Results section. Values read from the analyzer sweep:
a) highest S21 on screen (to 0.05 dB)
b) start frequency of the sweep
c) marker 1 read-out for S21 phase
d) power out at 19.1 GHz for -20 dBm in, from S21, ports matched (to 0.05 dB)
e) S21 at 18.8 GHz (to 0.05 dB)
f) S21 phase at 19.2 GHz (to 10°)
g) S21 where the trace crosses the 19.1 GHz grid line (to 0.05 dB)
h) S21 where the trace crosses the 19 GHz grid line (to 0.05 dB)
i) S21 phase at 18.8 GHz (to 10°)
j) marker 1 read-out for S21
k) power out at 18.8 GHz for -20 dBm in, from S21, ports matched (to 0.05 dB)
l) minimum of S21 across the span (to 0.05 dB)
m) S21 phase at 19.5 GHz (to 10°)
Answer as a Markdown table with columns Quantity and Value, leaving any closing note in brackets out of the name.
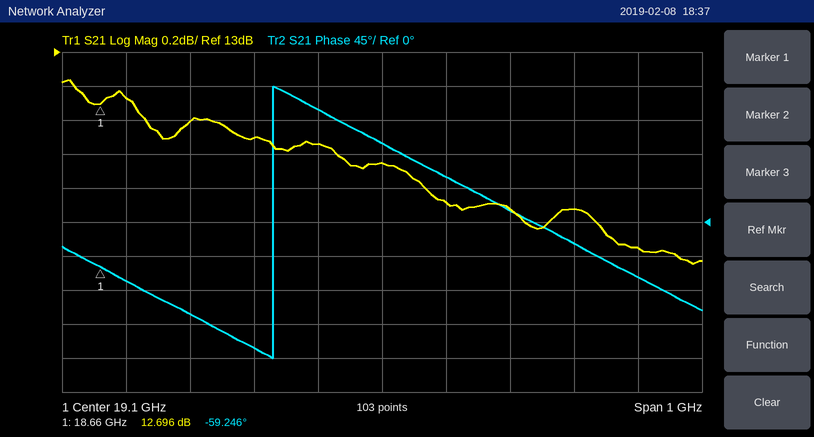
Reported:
| Quantity | Value |
|---|---|
| highest S21 on screen | 12.85 dB |
| start frequency of the sweep | 18.6 GHz |
| marker 1 read-out for S21 phase | -59.246° |
| power out at 19.1 GHz for -20 dBm in, from S21, ports matched | -7.65 dBm |
| S21 at 18.8 GHz | 12.60 dB |
| S21 phase at 19.2 GHz | 60° |
| S21 where the trace crosses the 19.1 GHz grid line | 12.35 dB |
| S21 where the trace crosses the 19 GHz grid line | 12.45 dB |
| S21 phase at 18.8 GHz | -120° |
| marker 1 read-out for S21 | 12.696 dB |
| power out at 18.8 GHz for -20 dBm in, from S21, ports matched | -7.40 dBm |
| minimum of S21 across the span | 11.75 dB |
| S21 phase at 19.5 GHz | -70° |
